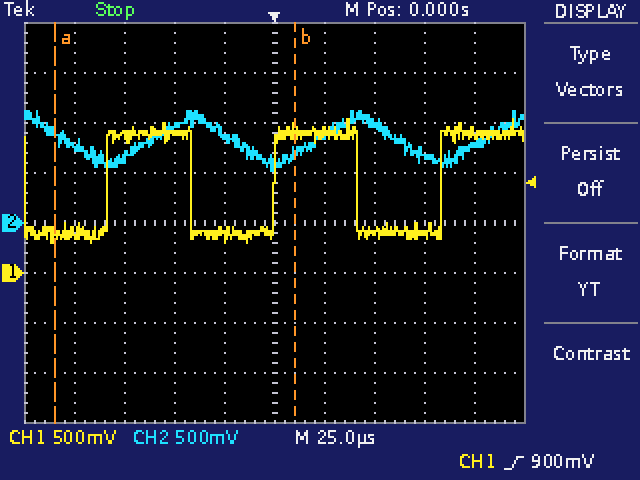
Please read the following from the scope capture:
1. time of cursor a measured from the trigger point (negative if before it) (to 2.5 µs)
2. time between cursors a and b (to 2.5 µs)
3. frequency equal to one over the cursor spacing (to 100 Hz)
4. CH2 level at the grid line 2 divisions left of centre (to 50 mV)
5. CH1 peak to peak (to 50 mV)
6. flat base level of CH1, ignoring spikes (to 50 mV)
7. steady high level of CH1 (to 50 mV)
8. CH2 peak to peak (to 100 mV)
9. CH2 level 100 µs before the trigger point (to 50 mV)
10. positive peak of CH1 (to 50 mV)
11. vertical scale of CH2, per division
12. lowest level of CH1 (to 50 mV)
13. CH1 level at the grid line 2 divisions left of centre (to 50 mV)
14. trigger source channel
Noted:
-110.0 µs
120.0 µs
8.3 kHz
950 mV
1.25 V
400 mV
1.40 V
600 mV
750 mV
1.55 V
500 mV
300 mV
1.40 V
CH1
